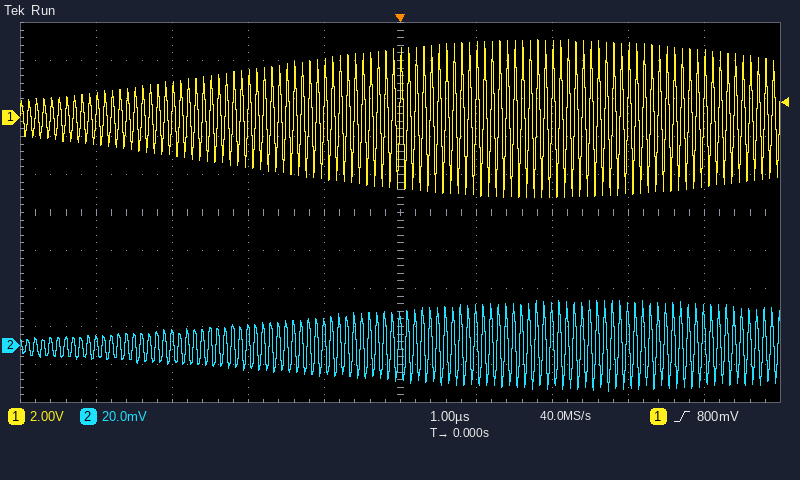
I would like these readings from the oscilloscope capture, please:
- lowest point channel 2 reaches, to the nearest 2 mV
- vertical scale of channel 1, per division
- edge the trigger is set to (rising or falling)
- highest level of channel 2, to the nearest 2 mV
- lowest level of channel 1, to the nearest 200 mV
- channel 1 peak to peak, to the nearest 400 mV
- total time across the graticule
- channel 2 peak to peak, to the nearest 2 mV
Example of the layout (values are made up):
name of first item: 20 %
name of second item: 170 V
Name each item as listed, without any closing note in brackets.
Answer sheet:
lowest point channel 2 reaches, to the nearest 2 mV: -24 mV
vertical scale of channel 1, per division: 2 V
edge the trigger is set to: rising
highest level of channel 2, to the nearest 2 mV: 24 mV
lowest level of channel 1, to the nearest 200 mV: -4.2 V
channel 1 peak to peak, to the nearest 400 mV: 8.4 V
total time across the graticule: 10 µs
channel 2 peak to peak, to the nearest 2 mV: 48 mV
